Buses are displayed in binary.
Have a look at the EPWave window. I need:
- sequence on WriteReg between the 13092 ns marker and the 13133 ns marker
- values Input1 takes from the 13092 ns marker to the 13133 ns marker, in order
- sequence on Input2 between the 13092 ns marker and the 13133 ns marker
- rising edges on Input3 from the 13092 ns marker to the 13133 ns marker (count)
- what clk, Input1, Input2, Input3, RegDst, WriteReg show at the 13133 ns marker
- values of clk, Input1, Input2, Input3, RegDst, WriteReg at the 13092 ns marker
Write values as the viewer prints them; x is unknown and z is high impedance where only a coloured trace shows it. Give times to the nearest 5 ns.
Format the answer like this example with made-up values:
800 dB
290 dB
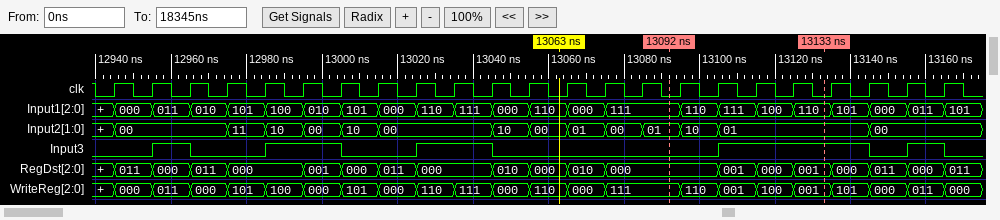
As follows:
111, 110, 001, 100, 001
111, 110, 111, 100, 110
01, 10, 01
1
clk=0, Input1=110, Input2=01, Input3=1, RegDst=001, WriteReg=001
clk=0, Input1=111, Input2=01, Input3=0, RegDst=000, WriteReg=111
